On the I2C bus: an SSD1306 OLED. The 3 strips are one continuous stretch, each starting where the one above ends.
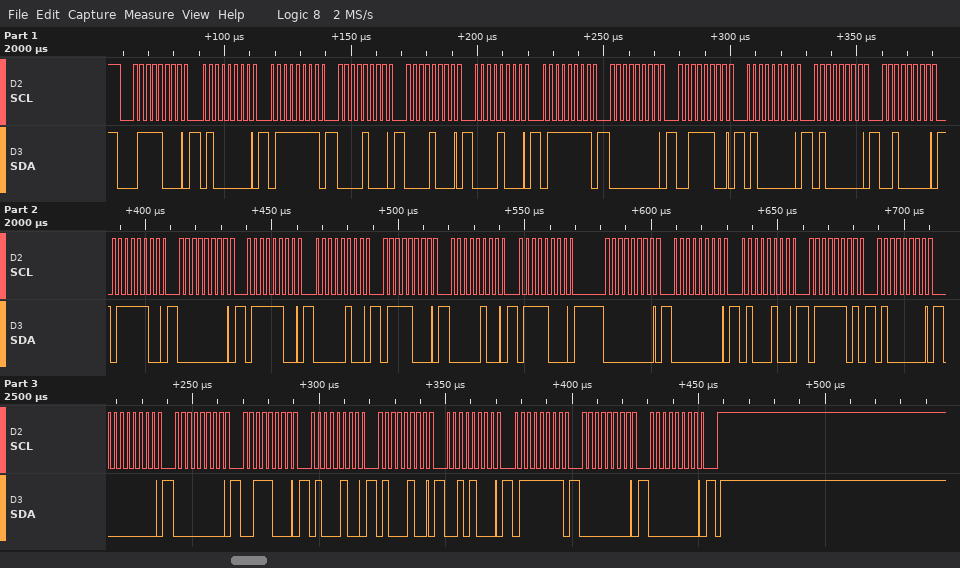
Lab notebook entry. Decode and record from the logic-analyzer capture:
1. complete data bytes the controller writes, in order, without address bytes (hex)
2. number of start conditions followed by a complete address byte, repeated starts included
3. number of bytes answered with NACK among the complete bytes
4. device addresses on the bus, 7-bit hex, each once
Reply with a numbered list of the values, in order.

1. 40 7F 08 08 08 7F 00 3C 40 40 20 7C 00 7C 04 78 04 78 00 00 44 7D 40 00 00 38 44 44 28 7F 00 00
2. 1
3. 0
4. 0x3C
